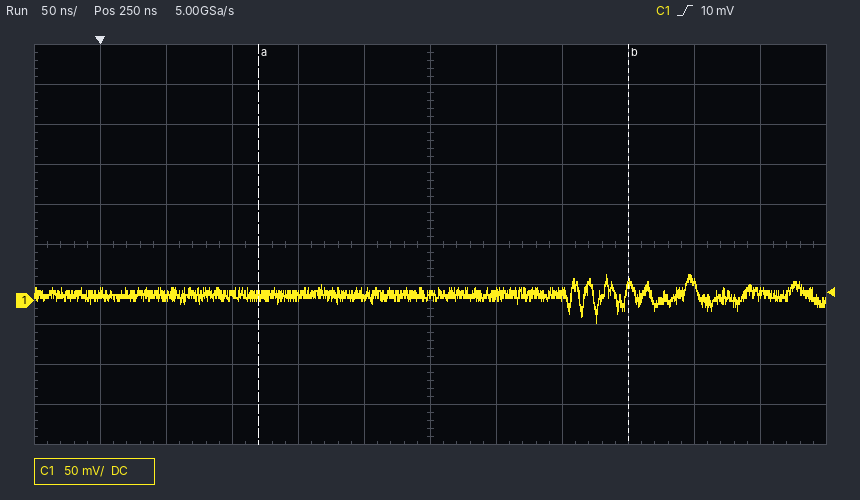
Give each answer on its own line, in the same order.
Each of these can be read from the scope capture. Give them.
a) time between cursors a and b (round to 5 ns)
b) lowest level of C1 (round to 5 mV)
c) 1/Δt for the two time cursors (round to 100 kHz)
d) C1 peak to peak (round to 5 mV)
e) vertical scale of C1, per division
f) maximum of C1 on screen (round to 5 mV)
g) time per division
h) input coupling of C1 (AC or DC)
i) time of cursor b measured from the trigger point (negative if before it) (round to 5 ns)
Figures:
280 ns
-30 mV
3.6 MHz
60 mV
50 mV
30 mV
50 ns
DC
+400 ns
